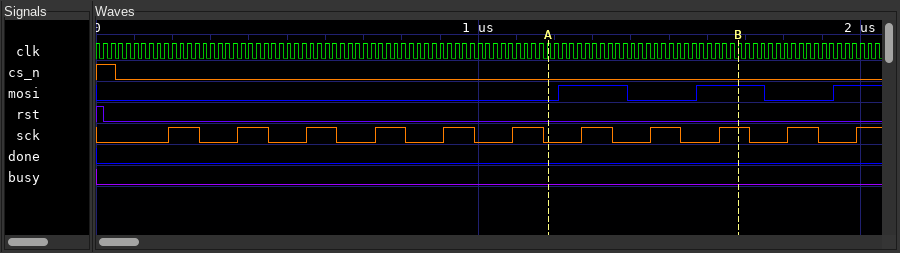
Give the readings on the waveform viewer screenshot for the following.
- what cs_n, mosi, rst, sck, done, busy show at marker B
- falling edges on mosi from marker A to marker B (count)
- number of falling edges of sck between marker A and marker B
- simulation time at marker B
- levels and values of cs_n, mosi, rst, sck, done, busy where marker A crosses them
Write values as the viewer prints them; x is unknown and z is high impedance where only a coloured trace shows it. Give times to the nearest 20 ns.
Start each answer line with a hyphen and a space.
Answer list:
- cs_n=0, mosi=1, rst=0, sck=1, done=0, busy=0
- 1
- 2
- 1680 ns
- cs_n=0, mosi=0, rst=0, sck=0, done=0, busy=0
